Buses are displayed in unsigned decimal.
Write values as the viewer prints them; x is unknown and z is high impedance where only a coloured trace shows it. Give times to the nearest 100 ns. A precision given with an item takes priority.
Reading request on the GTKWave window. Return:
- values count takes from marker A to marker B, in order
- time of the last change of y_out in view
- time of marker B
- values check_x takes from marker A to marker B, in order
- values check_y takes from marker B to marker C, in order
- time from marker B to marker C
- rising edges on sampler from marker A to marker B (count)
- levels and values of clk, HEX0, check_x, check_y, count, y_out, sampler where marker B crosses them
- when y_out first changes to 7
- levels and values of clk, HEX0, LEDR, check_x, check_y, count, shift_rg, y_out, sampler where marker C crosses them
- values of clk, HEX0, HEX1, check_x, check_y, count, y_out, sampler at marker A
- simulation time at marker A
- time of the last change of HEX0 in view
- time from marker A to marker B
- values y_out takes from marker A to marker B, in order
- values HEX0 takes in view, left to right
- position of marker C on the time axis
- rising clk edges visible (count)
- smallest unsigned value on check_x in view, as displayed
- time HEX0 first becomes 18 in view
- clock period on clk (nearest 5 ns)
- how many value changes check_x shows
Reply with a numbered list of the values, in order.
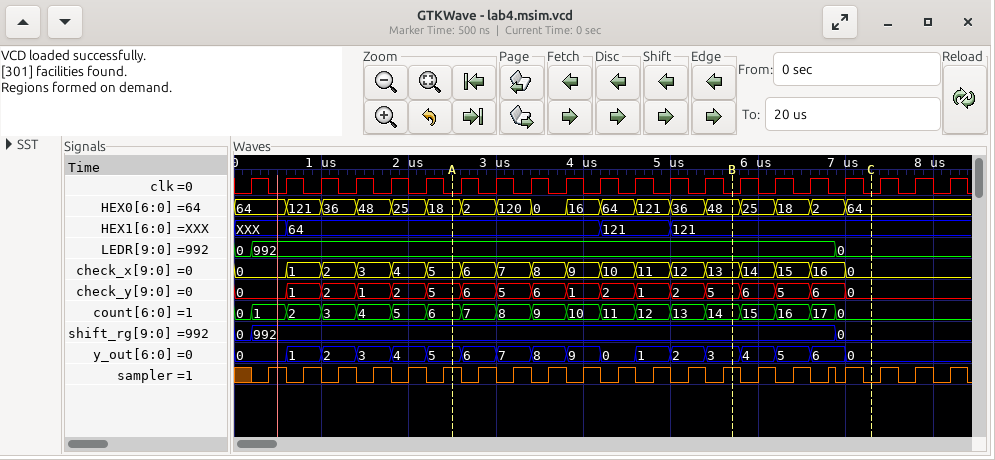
1. 6, 7, 8, 9, 10, 11, 12, 13, 14
2. 7000 ns
3. 5700 ns
4. 5, 6, 7, 8, 9, 10, 11, 12, 13
5. 5, 6, 5, 6, 0
6. 1600 ns
7. 8
8. clk=0, HEX0=48, check_x=13, check_y=5, count=14, y_out=3, sampler=1
9. 3000 ns
10. clk=0, HEX0=64, LEDR=0, check_x=0, check_y=0, count=0, shift_rg=0, y_out=0, sampler=0
11. clk=0, HEX0=18, HEX1=64, check_x=5, check_y=5, count=6, y_out=5, sampler=1
12. 2500 ns
13. 7000 ns
14. 3200 ns
15. 5, 6, 7, 8, 9, 0, 1, 2, 3
16. 64, 121, 36, 48, 25, 18, 2, 120, 0, 16, 64, 121, 36, 48, 25, 18, 2, 64
17. 7300 ns
18. 21
19. 0
20. 2200 ns
21. 400 ns
22. 17
